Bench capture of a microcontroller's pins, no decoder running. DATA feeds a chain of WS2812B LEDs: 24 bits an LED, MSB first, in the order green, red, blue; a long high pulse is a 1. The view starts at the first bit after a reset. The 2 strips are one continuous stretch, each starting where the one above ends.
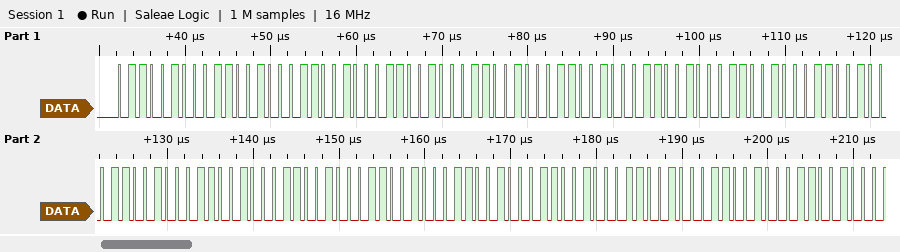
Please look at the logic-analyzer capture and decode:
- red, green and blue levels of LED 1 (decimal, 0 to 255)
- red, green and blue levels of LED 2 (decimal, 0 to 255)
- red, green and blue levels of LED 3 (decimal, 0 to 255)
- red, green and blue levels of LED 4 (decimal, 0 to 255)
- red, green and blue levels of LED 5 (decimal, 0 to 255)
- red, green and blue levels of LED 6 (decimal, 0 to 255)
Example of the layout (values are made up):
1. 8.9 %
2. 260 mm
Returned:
1. 100, 100, 100
2. 100, 100, 100
3. 100, 100, 100
4. 100, 100, 100
5. 100, 100, 100
6. 100, 100, 100
